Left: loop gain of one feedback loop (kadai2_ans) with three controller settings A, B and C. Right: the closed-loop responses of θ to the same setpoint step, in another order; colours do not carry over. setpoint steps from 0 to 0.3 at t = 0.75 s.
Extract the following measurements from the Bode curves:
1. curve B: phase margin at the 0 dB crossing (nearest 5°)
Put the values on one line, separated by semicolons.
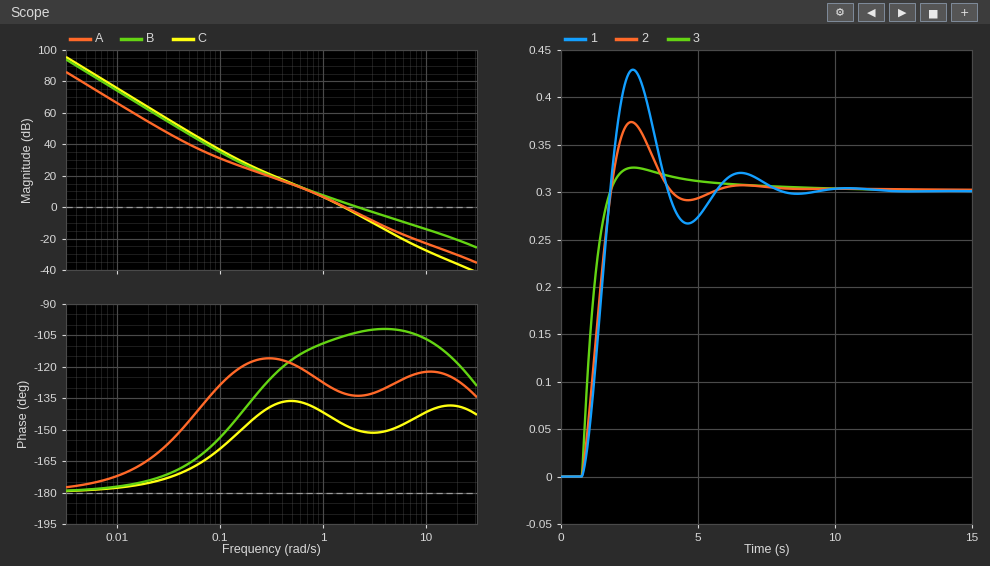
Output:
75°
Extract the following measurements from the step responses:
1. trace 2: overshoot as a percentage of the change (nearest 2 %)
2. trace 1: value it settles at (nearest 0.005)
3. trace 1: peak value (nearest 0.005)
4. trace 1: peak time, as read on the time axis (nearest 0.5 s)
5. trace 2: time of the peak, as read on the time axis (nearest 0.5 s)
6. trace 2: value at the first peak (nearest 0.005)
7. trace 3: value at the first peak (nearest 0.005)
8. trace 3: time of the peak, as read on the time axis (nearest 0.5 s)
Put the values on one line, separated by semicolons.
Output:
24 %; 0.300; 0.430; 2.5 s; 2.5 s; 0.375; 0.325; 2.5 s
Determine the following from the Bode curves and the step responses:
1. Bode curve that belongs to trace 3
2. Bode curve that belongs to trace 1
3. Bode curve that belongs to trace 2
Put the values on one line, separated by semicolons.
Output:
B; C; A
